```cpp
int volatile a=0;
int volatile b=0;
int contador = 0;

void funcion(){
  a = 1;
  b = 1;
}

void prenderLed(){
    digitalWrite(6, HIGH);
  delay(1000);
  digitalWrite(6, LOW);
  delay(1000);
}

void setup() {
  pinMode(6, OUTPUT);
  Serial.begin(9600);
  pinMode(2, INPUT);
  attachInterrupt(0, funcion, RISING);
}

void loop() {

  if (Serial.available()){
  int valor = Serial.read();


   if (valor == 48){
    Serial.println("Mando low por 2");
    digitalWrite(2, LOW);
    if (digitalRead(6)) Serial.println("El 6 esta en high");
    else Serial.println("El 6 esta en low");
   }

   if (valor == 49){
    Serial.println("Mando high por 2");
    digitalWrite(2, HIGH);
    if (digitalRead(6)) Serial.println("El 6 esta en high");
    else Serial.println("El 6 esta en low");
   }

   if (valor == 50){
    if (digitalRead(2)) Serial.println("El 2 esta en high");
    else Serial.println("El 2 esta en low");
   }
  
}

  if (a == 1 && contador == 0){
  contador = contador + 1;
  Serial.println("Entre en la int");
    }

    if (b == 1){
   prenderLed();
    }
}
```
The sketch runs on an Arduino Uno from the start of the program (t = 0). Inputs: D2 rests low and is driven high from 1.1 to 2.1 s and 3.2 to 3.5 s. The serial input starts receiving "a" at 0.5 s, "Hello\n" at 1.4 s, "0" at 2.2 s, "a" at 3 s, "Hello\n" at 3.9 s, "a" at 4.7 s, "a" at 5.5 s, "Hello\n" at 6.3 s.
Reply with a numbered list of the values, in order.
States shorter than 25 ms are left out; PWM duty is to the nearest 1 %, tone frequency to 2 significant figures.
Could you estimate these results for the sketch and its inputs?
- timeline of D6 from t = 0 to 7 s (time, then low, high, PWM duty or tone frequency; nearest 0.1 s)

1. 0 s low; 1.1 s high; 2.1 s low; 3.1 s high; 4.1 s low; 5.1 s high; 6.1 s low
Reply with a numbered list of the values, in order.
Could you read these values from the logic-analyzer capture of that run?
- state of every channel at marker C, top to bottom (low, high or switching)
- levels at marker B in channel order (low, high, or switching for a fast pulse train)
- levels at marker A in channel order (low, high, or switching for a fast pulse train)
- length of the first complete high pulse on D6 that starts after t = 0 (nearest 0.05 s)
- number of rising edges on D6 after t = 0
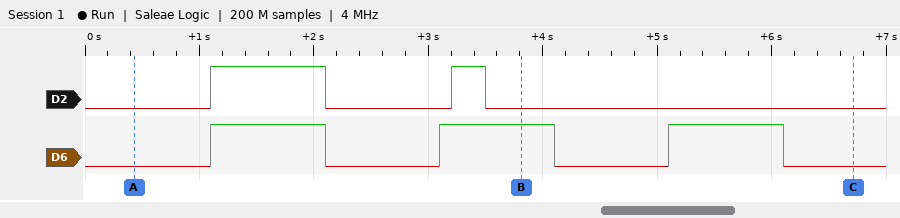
1. D2 low, D6 low
2. D2 low, D6 high
3. D2 low, D6 low
4. 1.00 s
5. 3
